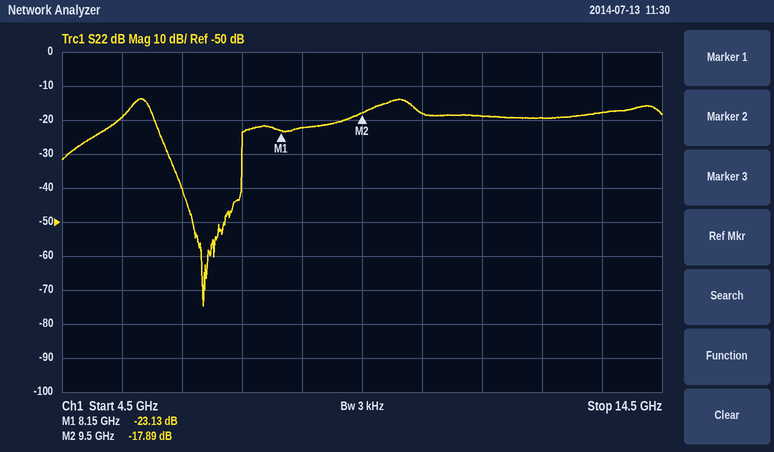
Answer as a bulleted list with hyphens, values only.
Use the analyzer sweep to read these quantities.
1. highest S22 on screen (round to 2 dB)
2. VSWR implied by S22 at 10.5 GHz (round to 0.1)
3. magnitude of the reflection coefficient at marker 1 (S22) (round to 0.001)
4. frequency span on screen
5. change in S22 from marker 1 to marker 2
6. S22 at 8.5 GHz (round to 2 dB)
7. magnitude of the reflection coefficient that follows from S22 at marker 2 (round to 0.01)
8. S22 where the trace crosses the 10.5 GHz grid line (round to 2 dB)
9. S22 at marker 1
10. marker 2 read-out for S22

- -14 dB
- 1.3
- 0.070
- 10 GHz
- 5.24 dB
- -22 dB
- 0.13
- -18 dB
- -23.13 dB
- -17.89 dB
